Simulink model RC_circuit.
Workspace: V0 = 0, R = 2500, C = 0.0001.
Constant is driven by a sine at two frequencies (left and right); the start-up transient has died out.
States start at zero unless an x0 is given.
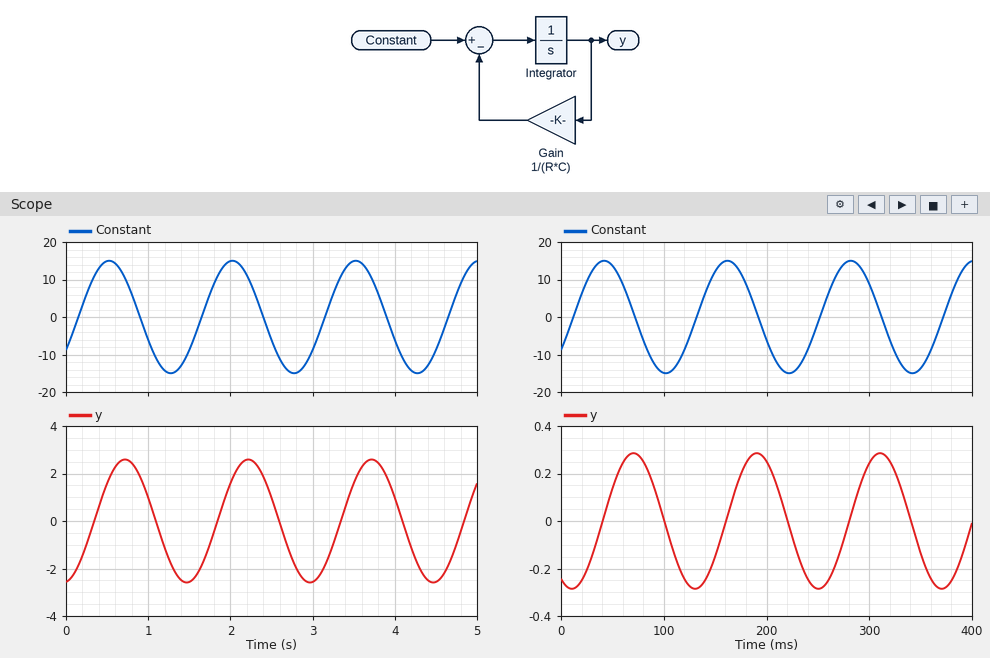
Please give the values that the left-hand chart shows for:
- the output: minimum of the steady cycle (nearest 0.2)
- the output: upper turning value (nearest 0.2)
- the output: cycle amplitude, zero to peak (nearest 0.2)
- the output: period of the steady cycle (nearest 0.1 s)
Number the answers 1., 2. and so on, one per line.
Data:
1. -2.6
2. 2.6
3. 2.6
4. 1.5 s
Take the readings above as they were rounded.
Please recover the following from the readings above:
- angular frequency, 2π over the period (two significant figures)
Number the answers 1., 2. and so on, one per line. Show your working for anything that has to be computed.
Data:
1. 2π / 1.5 = 4.2 rad/s
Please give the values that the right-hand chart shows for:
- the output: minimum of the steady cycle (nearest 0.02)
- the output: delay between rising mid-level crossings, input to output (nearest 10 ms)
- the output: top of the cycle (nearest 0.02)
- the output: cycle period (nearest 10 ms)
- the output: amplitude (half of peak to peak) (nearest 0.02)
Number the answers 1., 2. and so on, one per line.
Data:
1. -0.28
2. 30 ms
3. 0.28
4. 120 ms
5. 0.28
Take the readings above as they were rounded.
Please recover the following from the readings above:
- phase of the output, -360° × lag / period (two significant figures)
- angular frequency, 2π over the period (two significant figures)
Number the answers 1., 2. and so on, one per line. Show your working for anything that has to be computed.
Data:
1. -360 × 30 / 120 = -90°
2. 2π / 120 = 0.052 rad/ms
